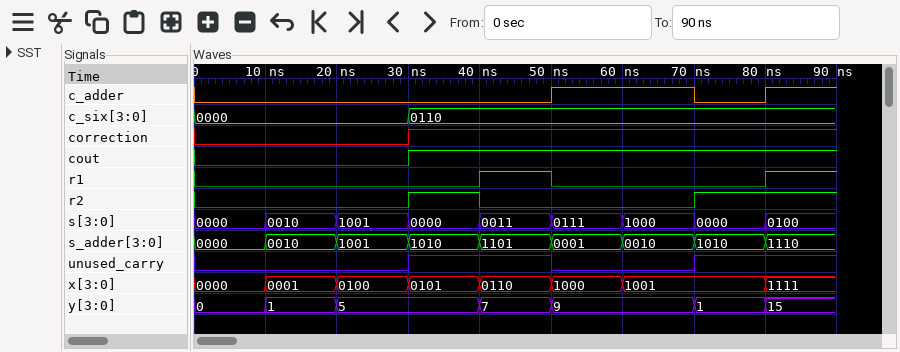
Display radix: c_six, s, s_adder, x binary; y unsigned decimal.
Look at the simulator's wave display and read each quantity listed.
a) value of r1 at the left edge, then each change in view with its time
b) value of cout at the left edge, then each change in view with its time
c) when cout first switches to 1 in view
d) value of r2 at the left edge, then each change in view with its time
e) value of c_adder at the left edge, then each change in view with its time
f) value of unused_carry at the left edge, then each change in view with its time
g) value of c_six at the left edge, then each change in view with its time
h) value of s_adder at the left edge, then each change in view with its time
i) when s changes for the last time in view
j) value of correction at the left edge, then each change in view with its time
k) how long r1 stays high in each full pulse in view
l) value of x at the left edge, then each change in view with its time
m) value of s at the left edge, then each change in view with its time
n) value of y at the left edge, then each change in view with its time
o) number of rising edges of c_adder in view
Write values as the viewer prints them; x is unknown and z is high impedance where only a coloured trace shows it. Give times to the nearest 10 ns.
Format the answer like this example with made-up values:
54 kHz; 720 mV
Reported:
0, 1 at 40 ns, 0 at 50 ns, 1 at 80 ns; 0, 1 at 30 ns; 30 ns; 0, 1 at 30 ns, 0 at 40 ns, 1 at 70 ns; 0, 1 at 50 ns, 0 at 70 ns, 1 at 80 ns; 0, 1 at 30 ns, 0 at 50 ns, 1 at 70 ns; 0000, 0110 at 30 ns; 0000, 0010 at 10 ns, 1001 at 20 ns, 1010 at 30 ns, 1101 at 40 ns, 0001 at 50 ns, 0010 at 60 ns, 1010 at 70 ns, 1110 at 80 ns; 80 ns; 0, 1 at 30 ns; 10 ns; 0000, 0001 at 10 ns, 0100 at 20 ns, 0101 at 30 ns, 0110 at 40 ns, 1000 at 50 ns, 1001 at 60 ns, 1111 at 80 ns; 0000, 0010 at 10 ns, 1001 at 20 ns, 0000 at 30 ns, 0011 at 40 ns, 0111 at 50 ns, 1000 at 60 ns, 0000 at 70 ns, 0100 at 80 ns; 0, 1 at 10 ns, 5 at 20 ns, 7 at 40 ns, 9 at 50 ns, 1 at 70 ns, 15 at 80 ns; 2
